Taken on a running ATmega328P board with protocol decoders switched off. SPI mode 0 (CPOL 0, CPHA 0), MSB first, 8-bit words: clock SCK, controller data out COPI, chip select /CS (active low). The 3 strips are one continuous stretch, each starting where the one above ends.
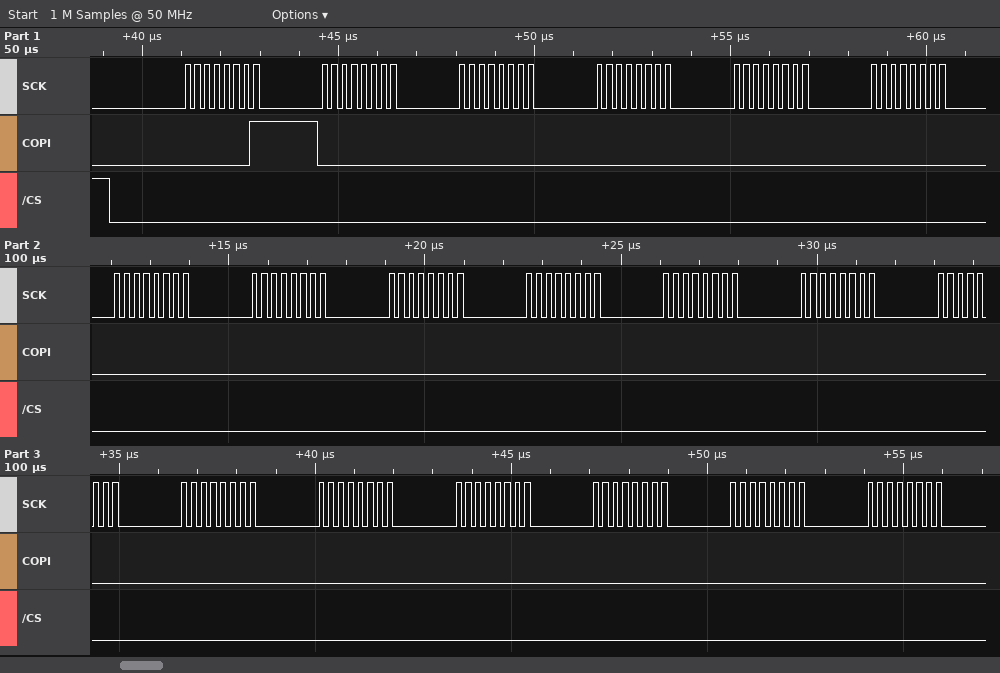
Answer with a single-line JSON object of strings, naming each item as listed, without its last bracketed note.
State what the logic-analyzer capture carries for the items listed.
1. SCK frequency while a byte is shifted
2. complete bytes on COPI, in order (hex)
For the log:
{"SCK frequency while a byte is shifted": "4 MHz", "complete bytes on COPI, in order": "0x01 0x00 0x00 0x00 0x00 0x00 0x00 0x00 0x00 0x00 0x00 0x00 0x00 0x00 0x00 0x00 0x00 0x00 0x00"}
